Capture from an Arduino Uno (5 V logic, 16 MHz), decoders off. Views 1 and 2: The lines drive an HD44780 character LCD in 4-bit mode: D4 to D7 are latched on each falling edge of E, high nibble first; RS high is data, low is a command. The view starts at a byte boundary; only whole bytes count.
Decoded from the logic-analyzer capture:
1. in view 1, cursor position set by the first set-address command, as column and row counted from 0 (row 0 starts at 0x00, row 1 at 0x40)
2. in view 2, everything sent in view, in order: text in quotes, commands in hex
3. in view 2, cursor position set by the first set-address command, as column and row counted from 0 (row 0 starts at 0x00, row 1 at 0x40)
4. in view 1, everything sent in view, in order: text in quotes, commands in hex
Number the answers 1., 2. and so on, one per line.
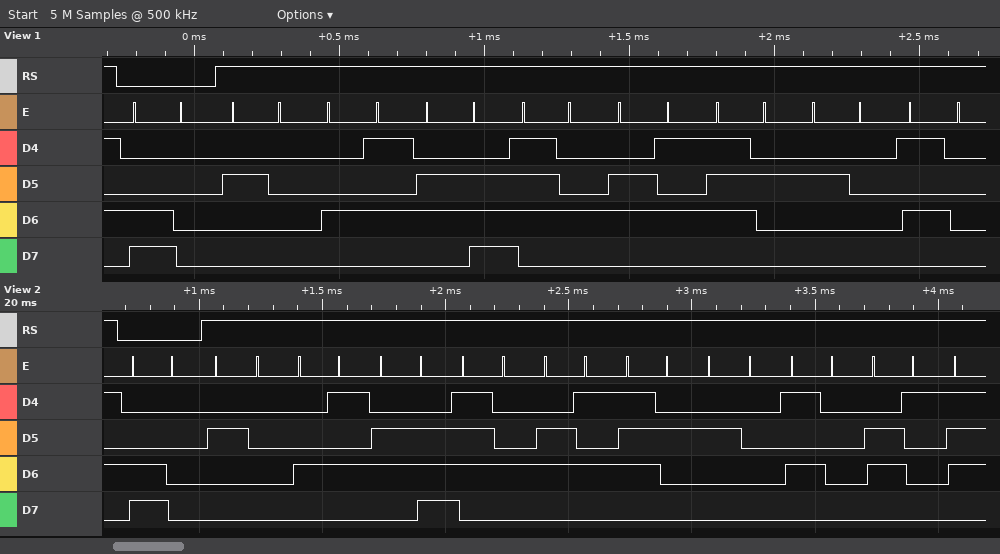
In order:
1. column 0, row 1
2. 0xC0 " Enter Pa"
3. column 0, row 1
4. 0xC0 " Enter P"
